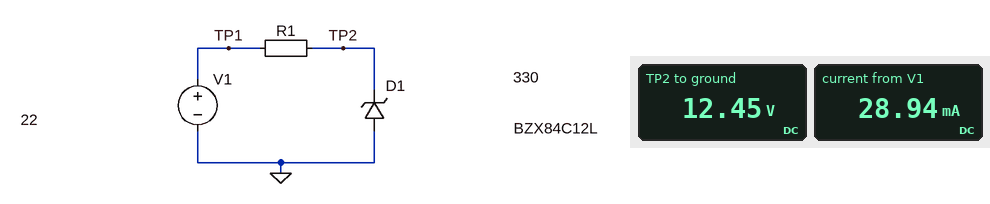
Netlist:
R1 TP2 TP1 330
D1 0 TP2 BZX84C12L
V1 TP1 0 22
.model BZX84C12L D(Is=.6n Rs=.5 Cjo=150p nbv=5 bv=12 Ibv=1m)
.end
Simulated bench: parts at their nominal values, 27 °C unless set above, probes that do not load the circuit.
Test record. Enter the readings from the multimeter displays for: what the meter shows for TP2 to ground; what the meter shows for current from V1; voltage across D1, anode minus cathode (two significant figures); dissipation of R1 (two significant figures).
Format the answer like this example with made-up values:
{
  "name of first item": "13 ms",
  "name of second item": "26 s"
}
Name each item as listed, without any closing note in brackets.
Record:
{
  "what the meter shows for TP2 to ground": "12.45 V",
  "what the meter shows for current from V1": "28.94 mA",
  "voltage across D1, anode minus cathode": "-12 V",
  "dissipation of R1": "280 mW"
}
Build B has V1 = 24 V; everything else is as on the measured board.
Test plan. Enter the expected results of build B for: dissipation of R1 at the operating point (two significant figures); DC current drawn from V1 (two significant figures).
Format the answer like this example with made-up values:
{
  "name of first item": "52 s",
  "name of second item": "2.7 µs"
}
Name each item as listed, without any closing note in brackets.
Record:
{
  "dissipation of R1 at the operating point": "400 mW",
  "DC current drawn from V1": "35 mA"
}
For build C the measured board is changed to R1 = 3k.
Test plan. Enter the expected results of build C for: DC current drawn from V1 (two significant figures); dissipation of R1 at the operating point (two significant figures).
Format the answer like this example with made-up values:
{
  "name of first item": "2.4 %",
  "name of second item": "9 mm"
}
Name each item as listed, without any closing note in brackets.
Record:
{
  "DC current drawn from V1": "3.3 mA",
  "dissipation of R1 at the operating point": "32 mW"
}
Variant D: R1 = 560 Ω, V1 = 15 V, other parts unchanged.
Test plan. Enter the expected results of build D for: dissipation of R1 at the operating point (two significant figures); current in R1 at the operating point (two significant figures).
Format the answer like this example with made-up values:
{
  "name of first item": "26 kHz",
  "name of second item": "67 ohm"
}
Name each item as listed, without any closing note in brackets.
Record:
{
  "dissipation of R1 at the operating point": "14 mW",
  "current in R1 at the operating point": "5.0 mA"
}
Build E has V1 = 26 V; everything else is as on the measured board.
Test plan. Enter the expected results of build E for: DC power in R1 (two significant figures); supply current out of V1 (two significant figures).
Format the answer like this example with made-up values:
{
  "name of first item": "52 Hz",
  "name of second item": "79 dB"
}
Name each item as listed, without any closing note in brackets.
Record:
{
  "DC power in R1": "550 mW",
  "supply current out of V1": "41 mA"
}
